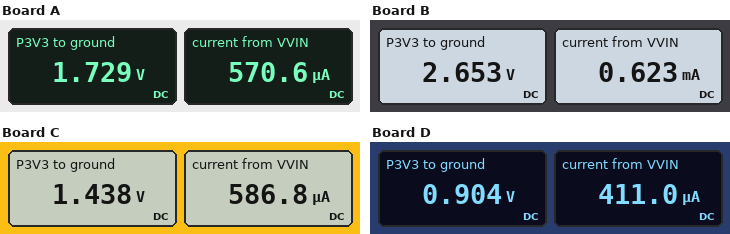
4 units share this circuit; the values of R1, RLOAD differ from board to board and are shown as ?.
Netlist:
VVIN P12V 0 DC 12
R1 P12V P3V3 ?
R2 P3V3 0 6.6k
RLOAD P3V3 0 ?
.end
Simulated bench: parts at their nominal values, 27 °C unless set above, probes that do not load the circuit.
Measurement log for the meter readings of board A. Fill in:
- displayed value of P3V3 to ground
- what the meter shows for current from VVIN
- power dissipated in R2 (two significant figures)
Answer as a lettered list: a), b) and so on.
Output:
a) 1.729 V
b) 570.6 µA
c) 450 µW
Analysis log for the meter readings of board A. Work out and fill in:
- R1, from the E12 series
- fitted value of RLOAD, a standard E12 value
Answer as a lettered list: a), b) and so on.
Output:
a) 18 kΩ
b) 5.6 kΩ
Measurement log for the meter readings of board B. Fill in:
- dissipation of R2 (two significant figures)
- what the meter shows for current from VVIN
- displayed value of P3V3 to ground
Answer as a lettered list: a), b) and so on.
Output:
a) 1.1 mW
b) 0.623 mA
c) 2.653 V
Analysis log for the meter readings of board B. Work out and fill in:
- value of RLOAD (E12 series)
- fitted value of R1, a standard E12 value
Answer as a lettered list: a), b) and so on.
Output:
a) 12 kΩ
b) 15 kΩ
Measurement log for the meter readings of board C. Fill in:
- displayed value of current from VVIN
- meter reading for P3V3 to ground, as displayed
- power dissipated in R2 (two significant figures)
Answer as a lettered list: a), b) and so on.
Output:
a) 586.8 µA
b) 1.438 V
c) 310 µW
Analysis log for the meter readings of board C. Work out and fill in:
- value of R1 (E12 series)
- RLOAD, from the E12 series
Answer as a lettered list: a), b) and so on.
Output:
a) 18 kΩ
b) 3.9 kΩ
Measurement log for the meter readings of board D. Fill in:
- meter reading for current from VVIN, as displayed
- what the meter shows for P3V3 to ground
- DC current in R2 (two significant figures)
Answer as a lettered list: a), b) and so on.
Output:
a) 411.0 µA
b) 0.904 V
c) 140 µA
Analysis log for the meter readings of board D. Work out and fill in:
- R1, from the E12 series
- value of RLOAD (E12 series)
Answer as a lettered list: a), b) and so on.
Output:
a) 27 kΩ
b) 3.3 kΩ
